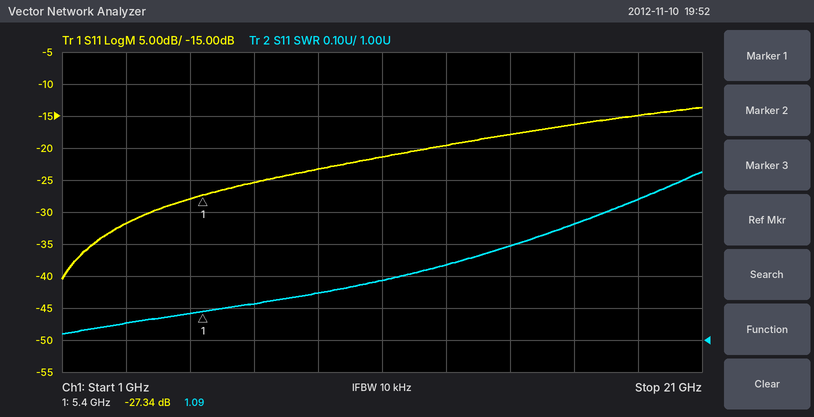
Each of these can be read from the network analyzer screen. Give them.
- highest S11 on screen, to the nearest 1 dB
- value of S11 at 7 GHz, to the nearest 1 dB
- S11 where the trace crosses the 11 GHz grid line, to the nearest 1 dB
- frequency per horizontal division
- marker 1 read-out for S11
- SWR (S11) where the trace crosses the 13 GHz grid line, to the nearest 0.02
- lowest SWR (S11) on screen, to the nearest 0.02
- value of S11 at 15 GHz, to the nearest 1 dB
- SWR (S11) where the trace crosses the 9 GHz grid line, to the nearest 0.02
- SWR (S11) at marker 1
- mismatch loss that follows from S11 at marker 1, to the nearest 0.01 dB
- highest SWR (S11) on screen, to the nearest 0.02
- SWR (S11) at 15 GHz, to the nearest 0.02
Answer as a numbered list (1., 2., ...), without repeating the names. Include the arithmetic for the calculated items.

1. -14 dB
2. -25 dB
3. -21 dB
4. 2 GHz
5. -27.34 dB
6. 1.24
7. 1.02
8. -18 dB
9. 1.14
10. 1.09
11. −10 log10(1 − 10^(-27.34/10)) ≈ 0.01 dB
12. 1.52
13. 1.30
